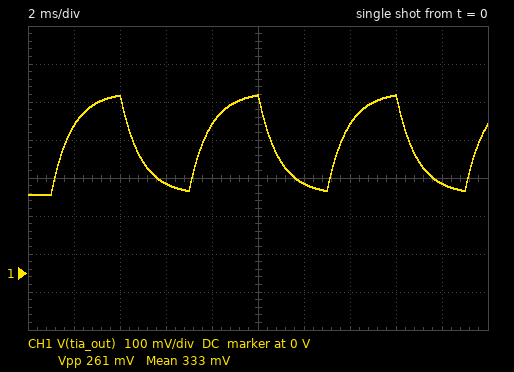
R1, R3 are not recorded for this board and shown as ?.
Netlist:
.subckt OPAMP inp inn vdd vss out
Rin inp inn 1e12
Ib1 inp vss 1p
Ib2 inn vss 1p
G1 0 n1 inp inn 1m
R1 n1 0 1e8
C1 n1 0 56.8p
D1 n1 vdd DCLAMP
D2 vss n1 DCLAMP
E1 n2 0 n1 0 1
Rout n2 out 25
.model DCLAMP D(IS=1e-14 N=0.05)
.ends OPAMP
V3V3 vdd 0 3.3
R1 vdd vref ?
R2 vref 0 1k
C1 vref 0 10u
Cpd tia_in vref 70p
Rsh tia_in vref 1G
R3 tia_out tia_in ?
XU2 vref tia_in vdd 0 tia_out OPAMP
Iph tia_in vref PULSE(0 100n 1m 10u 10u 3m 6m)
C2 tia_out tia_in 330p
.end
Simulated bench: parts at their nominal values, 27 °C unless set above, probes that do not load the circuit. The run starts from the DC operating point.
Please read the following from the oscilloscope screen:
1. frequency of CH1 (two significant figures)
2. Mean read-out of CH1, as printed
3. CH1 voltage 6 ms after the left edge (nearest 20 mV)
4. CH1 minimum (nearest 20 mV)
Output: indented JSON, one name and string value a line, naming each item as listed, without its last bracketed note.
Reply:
{
  "frequency of CH1": "170 Hz",
  "Mean read-out of CH1, as printed": "333 mV",
  "CH1 voltage 6 ms after the left edge": "240 mV",
  "CH1 minimum": "200 mV"
}
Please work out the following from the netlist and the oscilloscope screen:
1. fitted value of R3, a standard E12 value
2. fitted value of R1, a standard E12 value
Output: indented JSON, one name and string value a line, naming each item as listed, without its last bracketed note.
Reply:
{
  "fitted value of R3, a standard E12 value": "2.7 MΩ",
  "fitted value of R1, a standard E12 value": "15 kΩ"
}
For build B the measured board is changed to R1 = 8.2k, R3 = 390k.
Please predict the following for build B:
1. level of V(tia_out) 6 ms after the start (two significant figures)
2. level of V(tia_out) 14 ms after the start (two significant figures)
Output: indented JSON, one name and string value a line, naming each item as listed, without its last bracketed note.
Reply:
{
  "level of V(tia_out) 6 ms after the start": "360 mV",
  "level of V(tia_out) 14 ms after the start": "400 mV"
}
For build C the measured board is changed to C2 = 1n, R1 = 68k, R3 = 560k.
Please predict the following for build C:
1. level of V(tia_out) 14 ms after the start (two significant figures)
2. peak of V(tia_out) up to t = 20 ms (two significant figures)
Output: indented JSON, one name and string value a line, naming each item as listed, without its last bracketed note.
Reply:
{
  "level of V(tia_out) 14 ms after the start": "94 mV",
  "peak of V(tia_out) up to t = 20 ms": "100 mV"
}
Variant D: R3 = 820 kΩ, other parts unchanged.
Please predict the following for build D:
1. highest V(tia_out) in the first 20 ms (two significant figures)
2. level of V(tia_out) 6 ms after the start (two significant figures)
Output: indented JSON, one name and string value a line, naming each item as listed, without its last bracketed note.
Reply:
{
  "highest V(tia_out) in the first 20 ms": "290 mV",
  "level of V(tia_out) 6 ms after the start": "210 mV"
}
